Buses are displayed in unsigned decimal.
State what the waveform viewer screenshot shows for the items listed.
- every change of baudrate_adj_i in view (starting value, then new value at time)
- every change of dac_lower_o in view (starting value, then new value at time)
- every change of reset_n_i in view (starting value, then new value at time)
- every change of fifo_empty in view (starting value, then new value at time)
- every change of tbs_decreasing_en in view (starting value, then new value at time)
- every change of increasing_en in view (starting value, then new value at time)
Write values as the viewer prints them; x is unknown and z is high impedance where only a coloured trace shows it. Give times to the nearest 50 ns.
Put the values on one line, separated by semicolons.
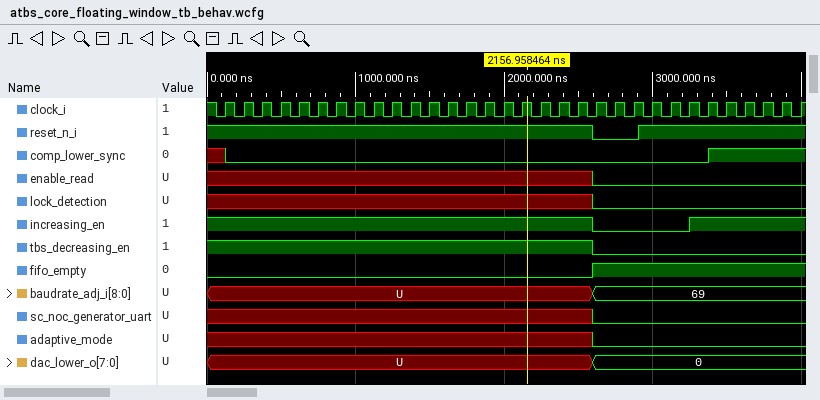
U, 69 at 2600 ns; U, 0 at 2600 ns; 1, 0 at 2600 ns, 1 at 2900 ns; 0, 1 at 2600 ns; 1, 0 at 2600 ns; 1, 0 at 2600 ns, 1 at 3250 ns
